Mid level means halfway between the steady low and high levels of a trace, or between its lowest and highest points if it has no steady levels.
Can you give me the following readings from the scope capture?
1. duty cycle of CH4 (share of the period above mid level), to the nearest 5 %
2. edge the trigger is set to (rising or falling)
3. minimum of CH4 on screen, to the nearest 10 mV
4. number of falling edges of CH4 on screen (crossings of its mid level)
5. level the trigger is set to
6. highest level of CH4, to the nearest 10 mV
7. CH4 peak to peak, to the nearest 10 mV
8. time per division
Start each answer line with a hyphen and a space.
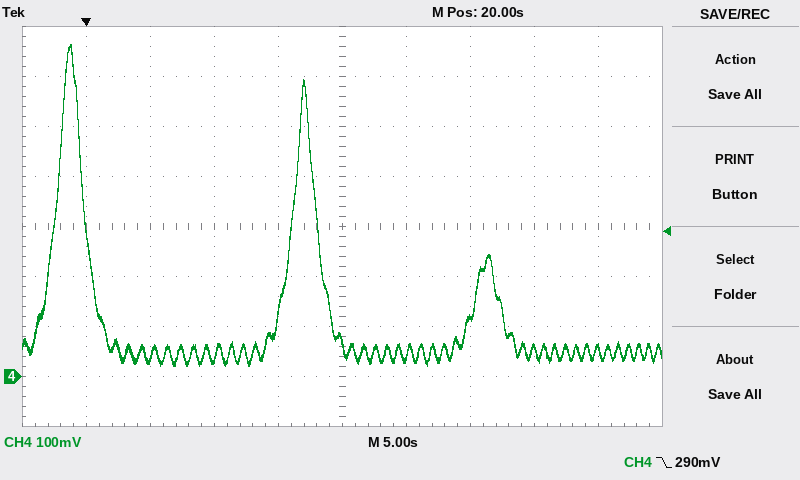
- 10 %
- falling
- 20 mV
- 2
- 290 mV
- 660 mV
- 640 mV
- 5 s
